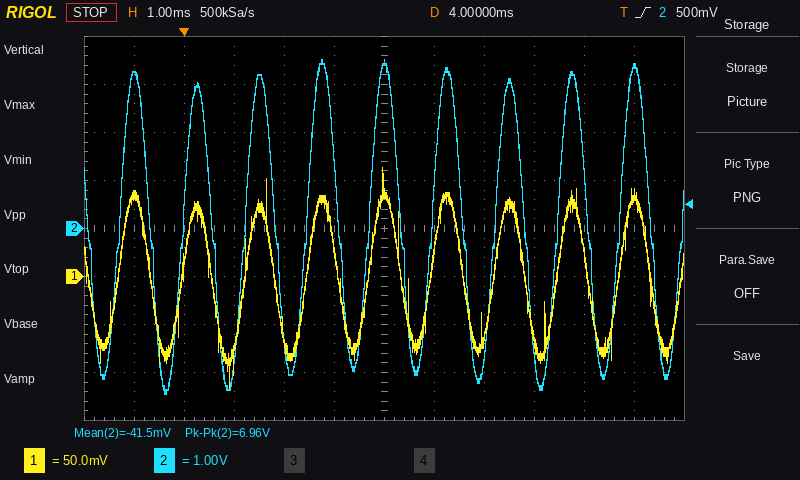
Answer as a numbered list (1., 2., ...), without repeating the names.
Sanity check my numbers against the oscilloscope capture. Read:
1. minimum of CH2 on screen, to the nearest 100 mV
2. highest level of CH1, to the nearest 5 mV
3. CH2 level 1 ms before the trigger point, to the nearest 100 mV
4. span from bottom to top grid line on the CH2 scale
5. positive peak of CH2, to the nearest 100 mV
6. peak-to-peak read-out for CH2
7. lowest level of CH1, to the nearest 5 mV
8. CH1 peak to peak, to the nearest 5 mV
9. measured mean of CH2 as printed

1. -3.4 V
2. 115 mV
3. 3.2 V
4. 8 V
5. 3.5 V
6. 6.96 V
7. -115 mV
8. 230 mV
9. -41.5 mV
